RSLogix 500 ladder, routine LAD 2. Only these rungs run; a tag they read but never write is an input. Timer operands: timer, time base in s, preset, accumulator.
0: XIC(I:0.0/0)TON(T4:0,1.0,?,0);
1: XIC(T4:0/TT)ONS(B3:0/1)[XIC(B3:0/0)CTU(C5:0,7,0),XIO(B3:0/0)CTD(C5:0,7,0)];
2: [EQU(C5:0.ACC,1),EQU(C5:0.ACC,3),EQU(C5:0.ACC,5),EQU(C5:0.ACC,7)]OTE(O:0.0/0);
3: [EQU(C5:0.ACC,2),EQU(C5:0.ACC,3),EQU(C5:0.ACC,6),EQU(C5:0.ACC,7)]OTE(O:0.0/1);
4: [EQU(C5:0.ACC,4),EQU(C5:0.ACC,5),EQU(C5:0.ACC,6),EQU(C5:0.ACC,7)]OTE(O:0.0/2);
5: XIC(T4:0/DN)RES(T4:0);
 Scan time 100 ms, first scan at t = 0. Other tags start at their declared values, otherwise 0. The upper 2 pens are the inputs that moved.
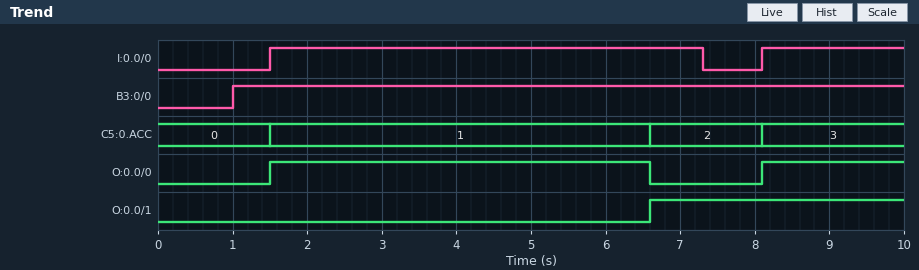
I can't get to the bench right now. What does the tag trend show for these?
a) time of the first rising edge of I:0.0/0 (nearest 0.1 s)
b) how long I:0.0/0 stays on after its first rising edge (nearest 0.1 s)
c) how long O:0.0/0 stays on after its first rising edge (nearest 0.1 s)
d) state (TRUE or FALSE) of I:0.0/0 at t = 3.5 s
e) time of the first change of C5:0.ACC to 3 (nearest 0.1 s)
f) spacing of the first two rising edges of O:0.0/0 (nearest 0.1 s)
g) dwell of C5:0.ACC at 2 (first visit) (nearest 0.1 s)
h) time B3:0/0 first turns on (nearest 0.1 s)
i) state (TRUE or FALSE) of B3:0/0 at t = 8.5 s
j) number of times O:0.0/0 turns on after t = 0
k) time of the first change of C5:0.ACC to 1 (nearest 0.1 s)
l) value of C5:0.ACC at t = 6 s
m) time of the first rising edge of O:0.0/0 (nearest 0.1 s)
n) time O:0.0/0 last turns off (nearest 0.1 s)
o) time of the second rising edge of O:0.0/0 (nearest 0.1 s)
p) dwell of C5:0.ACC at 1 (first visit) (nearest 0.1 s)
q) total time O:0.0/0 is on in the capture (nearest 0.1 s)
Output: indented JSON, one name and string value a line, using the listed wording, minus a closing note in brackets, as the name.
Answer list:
{
  "time of the first rising edge of I:0.0/0": "1.5 s",
  "how long I:0.0/0 stays on after its first rising edge": "5.8 s",
  "how long O:0.0/0 stays on after its first rising edge": "5.1 s",
  "state (TRUE or FALSE) of I:0.0/0 at t = 3.5 s": "TRUE",
  "time of the first change of C5:0.ACC to 3": "8.1 s",
  "spacing of the first two rising edges of O:0.0/0": "6.6 s",
  "dwell of C5:0.ACC at 2 (first visit)": "1.5 s",
  "time B3:0/0 first turns on": "1.0 s",
  "state (TRUE or FALSE) of B3:0/0 at t = 8.5 s": "TRUE",
  "number of times O:0.0/0 turns on after t = 0": "2",
  "time of the first change of C5:0.ACC to 1": "1.5 s",
  "value of C5:0.ACC at t = 6 s": "1",
  "time of the first rising edge of O:0.0/0": "1.5 s",
  "time O:0.0/0 last turns off": "6.6 s",
  "time of the second rising edge of O:0.0/0": "8.1 s",
  "dwell of C5:0.ACC at 1 (first visit)": "5.1 s",
  "total time O:0.0/0 is on in the capture": "7.0 s"
}
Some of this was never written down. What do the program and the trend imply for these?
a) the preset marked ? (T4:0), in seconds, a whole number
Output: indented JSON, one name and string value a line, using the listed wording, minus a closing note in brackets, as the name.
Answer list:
{
  "the preset marked ? (T4:0), in seconds, a whole number": "5 s"
}
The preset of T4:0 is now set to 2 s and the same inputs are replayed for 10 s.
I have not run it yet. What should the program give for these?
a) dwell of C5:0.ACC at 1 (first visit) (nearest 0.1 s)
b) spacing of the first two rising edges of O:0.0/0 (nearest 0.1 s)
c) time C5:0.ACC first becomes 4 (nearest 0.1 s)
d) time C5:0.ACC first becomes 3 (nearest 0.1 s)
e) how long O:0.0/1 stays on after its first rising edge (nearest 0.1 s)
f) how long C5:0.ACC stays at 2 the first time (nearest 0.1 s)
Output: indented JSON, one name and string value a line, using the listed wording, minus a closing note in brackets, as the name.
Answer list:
{
  "dwell of C5:0.ACC at 1 (first visit)": "2.1 s",
  "spacing of the first two rising edges of O:0.0/0": "4.2 s",
  "time C5:0.ACC first becomes 4": "8.1 s",
  "time C5:0.ACC first becomes 3": "5.7 s",
  "how long O:0.0/1 stays on after its first rising edge": "4.5 s",
  "how long C5:0.ACC stays at 2 the first time": "2.1 s"
}
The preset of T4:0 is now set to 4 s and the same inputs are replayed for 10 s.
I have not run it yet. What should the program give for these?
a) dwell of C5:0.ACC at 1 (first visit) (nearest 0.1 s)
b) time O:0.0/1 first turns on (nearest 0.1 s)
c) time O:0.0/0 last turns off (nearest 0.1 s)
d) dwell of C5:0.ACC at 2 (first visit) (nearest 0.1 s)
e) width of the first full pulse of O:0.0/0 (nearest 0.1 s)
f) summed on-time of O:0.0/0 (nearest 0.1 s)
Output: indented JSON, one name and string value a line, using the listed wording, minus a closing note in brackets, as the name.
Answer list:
{
  "dwell of C5:0.ACC at 1 (first visit)": "4.1 s",
  "time O:0.0/1 first turns on": "5.6 s",
  "time O:0.0/0 last turns off": "5.6 s",
  "dwell of C5:0.ACC at 2 (first visit)": "2.5 s",
  "width of the first full pulse of O:0.0/0": "4.1 s",
  "summed on-time of O:0.0/0": "6.0 s"
}
